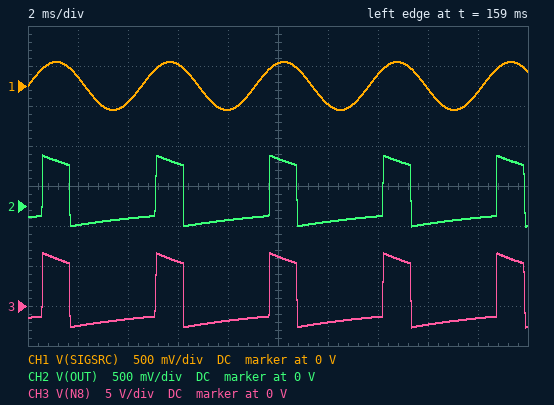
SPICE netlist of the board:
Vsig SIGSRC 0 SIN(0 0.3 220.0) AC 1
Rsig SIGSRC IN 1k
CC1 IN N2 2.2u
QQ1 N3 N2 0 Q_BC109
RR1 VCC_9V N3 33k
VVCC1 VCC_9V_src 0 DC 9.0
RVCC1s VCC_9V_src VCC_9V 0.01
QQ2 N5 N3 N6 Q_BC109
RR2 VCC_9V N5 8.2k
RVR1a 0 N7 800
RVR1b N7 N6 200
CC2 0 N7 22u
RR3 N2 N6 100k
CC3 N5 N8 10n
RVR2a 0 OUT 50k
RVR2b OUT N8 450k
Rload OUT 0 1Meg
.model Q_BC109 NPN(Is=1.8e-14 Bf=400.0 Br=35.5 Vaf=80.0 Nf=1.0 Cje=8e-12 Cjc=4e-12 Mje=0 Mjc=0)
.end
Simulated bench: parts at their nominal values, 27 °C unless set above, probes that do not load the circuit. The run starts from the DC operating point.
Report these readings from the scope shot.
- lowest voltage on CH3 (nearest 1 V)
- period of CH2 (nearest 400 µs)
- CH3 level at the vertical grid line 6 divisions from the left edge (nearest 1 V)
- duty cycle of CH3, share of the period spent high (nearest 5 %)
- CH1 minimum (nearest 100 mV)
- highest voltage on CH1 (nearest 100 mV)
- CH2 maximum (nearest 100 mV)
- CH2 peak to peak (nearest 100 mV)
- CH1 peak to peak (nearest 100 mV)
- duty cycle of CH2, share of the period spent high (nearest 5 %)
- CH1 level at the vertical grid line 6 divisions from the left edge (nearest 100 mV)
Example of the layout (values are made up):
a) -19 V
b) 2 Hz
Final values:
a) -3 V
b) 4.4 ms
c) -2 V
d) 25 %
e) -300 mV
f) 300 mV
g) 600 mV
h) 900 mV
i) 600 mV
j) 25 %
k) -200 mV
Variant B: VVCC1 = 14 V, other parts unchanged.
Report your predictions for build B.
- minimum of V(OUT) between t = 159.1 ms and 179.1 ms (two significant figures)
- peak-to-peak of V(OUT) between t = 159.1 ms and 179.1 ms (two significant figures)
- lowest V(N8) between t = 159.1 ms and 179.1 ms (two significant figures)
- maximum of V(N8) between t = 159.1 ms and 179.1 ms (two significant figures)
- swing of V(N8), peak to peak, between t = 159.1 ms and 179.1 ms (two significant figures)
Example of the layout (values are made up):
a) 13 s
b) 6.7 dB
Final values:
a) -450 mV
b) 1.4 V
c) -4.7 V
d) 10 V
e) 15 V
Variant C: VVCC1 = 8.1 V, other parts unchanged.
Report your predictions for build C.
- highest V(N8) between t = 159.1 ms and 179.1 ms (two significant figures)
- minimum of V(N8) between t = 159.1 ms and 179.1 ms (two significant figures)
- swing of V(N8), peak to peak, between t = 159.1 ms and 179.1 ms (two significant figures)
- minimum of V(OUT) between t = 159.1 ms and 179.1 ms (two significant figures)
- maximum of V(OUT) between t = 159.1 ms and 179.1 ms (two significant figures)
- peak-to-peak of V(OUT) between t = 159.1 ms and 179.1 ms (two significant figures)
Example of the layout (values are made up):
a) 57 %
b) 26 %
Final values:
a) 6.0 V
b) -2.4 V
c) 8.3 V
d) -230 mV
e) 570 mV
f) 800 mV
